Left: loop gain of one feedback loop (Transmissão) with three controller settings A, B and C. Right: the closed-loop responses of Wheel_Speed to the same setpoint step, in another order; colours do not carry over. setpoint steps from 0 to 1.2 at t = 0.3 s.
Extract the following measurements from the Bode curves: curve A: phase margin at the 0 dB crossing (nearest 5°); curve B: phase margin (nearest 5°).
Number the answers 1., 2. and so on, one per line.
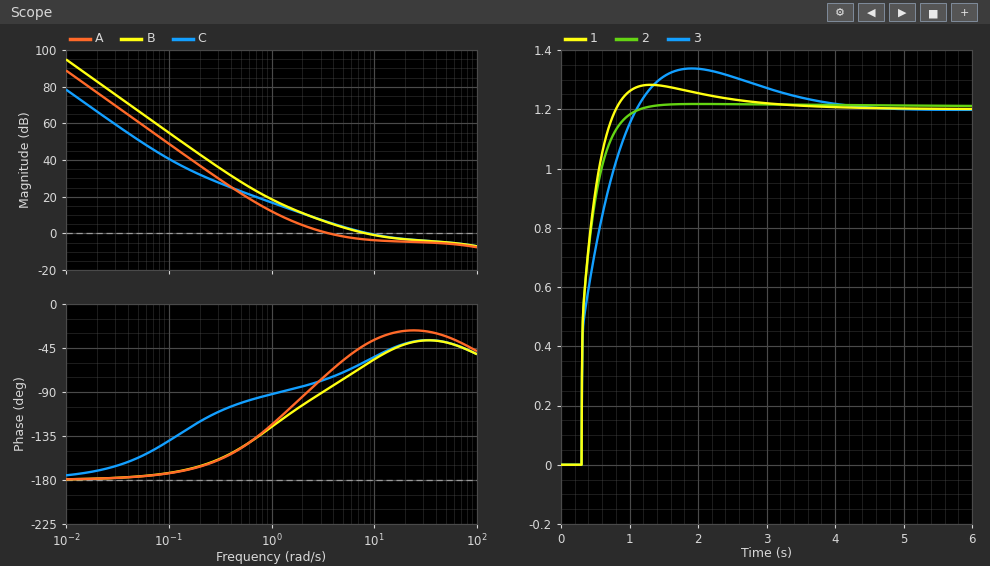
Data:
1. 110°
2. 120°
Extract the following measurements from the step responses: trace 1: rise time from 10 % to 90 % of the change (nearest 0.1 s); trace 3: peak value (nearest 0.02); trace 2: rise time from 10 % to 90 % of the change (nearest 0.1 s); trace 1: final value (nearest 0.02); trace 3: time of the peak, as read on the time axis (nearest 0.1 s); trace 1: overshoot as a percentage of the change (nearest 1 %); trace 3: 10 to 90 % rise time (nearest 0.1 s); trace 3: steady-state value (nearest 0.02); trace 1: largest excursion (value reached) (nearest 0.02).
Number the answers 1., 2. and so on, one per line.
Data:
1. 0.3 s
2. 1.34
3. 0.4 s
4. 1.20
5. 1.9 s
6. 7 %
7. 0.6 s
8. 1.20
9. 1.28
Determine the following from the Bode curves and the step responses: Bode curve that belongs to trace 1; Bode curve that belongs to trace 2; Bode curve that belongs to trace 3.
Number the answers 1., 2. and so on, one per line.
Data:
1. B
2. C
3. A
